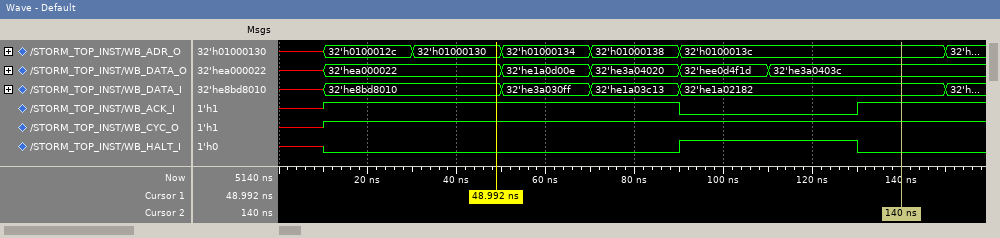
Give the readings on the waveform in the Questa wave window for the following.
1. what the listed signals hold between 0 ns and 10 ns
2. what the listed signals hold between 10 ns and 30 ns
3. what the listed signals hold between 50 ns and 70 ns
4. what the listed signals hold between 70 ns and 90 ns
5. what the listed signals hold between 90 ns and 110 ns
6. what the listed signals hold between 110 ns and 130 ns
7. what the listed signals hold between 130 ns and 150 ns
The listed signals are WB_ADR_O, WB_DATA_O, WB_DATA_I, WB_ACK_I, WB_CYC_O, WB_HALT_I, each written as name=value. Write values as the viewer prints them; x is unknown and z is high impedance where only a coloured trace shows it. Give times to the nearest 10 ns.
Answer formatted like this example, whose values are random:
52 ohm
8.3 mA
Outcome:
WB_ADR_O=x, WB_DATA_O=x, WB_DATA_I=x, WB_ACK_I=x, WB_CYC_O=x, WB_HALT_I=x
WB_ADR_O=32'h0100012c, WB_DATA_O=32'hea000022, WB_DATA_I=32'he8bd8010, WB_ACK_I=1, WB_CYC_O=1, WB_HALT_I=0
WB_ADR_O=32'h01000134, WB_DATA_O=32'he1a0d00e, WB_DATA_I=32'he3a030ff, WB_ACK_I=1, WB_CYC_O=1, WB_HALT_I=0
WB_ADR_O=32'h01000138, WB_DATA_O=32'he3a04020, WB_DATA_I=32'he1a03c13, WB_ACK_I=1, WB_CYC_O=1, WB_HALT_I=0
WB_ADR_O=32'h0100013c, WB_DATA_O=32'hee0d4f1d, WB_DATA_I=32'he1a02182, WB_ACK_I=0, WB_CYC_O=1, WB_HALT_I=1
WB_ADR_O=32'h0100013c, WB_DATA_O=32'he3a0403c, WB_DATA_I=32'he1a02182, WB_ACK_I=0, WB_CYC_O=1, WB_HALT_I=1
WB_ADR_O=32'h0100013c, WB_DATA_O=32'he3a0403c, WB_DATA_I=32'he1a02182, WB_ACK_I=1, WB_CYC_O=1, WB_HALT_I=0
